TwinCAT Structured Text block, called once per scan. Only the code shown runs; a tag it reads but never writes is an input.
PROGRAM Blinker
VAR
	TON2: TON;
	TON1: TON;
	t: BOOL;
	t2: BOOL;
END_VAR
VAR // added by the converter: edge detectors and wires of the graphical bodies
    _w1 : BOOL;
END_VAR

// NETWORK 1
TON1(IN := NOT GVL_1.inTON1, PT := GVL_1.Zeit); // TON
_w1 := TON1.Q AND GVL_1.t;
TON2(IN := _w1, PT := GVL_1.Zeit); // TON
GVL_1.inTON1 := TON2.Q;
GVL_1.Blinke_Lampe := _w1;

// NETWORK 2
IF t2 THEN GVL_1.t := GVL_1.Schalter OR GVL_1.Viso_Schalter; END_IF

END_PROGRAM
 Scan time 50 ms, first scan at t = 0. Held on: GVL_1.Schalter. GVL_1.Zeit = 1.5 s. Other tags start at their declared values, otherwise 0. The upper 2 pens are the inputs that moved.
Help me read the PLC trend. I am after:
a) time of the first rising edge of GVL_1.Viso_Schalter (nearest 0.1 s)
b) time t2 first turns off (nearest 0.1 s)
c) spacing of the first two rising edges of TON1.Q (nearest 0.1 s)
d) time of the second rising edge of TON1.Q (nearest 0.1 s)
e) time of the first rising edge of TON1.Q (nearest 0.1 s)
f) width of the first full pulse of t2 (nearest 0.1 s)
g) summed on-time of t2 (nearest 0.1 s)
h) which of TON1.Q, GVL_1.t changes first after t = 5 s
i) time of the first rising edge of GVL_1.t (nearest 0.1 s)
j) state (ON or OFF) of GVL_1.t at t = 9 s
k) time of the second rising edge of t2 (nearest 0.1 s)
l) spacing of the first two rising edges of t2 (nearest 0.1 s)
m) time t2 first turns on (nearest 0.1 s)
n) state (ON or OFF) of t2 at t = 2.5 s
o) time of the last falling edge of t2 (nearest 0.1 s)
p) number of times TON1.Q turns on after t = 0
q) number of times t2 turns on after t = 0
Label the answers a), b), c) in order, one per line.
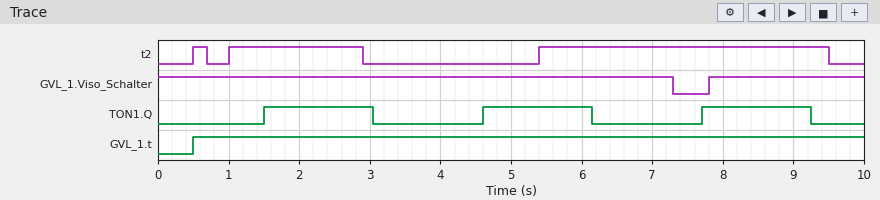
a) 7.8 s
b) 0.7 s
c) 3.1 s
d) 4.6 s
e) 1.5 s
f) 0.2 s
g) 6.2 s
h) TON1.Q
i) 0.5 s
j) ON
k) 1.0 s
l) 0.5 s
m) 0.5 s
n) ON
o) 9.5 s
p) 3
q) 3
